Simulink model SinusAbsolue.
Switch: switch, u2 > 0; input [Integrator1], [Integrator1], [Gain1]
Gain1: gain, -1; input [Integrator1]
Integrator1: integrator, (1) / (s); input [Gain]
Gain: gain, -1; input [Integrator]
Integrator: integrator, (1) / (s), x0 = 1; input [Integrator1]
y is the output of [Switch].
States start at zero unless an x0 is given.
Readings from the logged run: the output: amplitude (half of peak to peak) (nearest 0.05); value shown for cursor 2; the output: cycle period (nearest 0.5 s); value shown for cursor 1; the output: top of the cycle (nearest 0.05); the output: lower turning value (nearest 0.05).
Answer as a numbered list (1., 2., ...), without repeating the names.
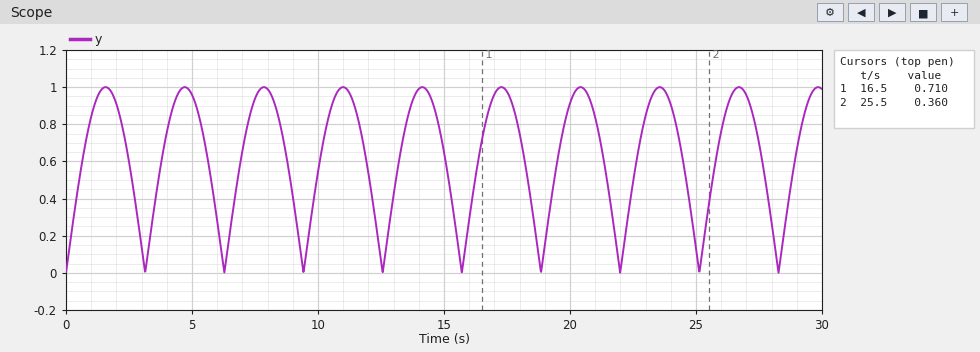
1. 0.50
2. 0.360
3. 3.0 s
4. 0.710
5. 1.00
6. 0.00
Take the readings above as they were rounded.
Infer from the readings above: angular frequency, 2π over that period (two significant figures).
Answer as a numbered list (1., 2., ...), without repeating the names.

1. 2.1 rad/s
